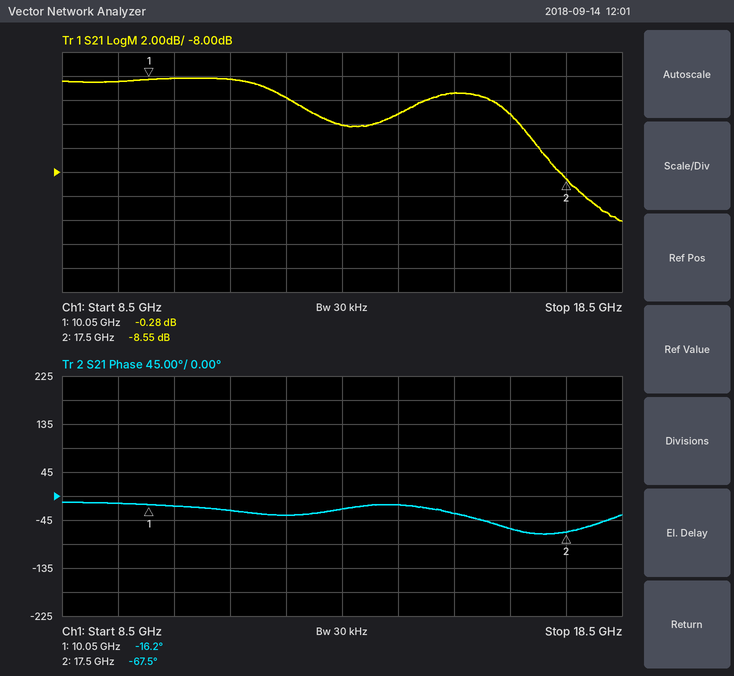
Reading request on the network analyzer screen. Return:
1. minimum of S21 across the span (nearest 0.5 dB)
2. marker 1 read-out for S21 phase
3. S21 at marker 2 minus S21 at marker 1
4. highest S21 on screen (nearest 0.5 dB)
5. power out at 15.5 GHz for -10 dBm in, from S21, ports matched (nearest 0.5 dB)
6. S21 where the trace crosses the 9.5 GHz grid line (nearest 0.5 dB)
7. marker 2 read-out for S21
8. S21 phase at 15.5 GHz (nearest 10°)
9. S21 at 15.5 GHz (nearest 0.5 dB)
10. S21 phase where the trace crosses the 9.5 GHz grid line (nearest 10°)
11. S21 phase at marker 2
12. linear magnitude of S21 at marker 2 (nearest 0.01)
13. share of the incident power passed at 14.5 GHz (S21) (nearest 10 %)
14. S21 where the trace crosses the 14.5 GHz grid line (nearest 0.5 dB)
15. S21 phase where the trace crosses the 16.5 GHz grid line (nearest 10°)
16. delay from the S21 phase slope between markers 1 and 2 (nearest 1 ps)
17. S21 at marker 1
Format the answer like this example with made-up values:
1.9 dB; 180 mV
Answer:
-12.0 dB; -16.2°; -8.27 dB; 0.0 dB; -11.5 dBm; -0.5 dB; -8.55 dB; -30°; -1.5 dB; -10°; -67.5°; 0.37; 50 %; -3.0 dB; -60°; 19 ps; -0.28 dB
